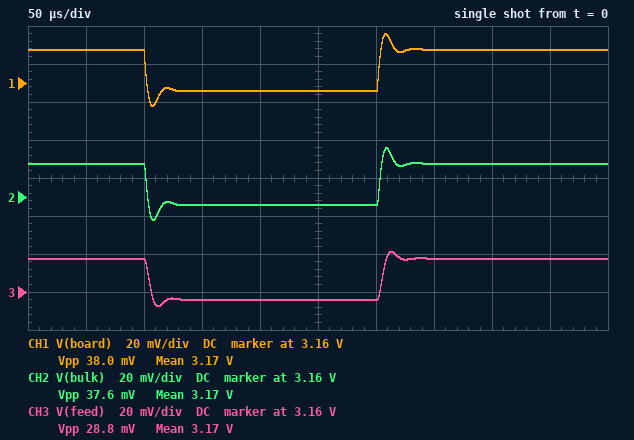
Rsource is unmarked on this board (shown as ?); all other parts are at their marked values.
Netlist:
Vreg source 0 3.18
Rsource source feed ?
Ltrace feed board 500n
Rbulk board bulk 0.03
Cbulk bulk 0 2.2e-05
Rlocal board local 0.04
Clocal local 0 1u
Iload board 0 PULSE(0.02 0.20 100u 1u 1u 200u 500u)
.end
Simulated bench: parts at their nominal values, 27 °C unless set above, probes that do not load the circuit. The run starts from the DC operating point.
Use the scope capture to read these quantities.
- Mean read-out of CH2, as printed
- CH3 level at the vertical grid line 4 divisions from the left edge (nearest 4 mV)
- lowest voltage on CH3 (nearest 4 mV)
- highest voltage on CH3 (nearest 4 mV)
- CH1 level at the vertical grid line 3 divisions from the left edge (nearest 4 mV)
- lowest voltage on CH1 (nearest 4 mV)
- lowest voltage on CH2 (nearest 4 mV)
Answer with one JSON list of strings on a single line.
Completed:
["3.17 V", "3.156 V", "3.152 V", "3.180 V", "3.156 V", "3.148 V", "3.148 V"]
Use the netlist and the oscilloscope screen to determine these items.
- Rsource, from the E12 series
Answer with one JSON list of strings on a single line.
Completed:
["0.12 Ω"]
